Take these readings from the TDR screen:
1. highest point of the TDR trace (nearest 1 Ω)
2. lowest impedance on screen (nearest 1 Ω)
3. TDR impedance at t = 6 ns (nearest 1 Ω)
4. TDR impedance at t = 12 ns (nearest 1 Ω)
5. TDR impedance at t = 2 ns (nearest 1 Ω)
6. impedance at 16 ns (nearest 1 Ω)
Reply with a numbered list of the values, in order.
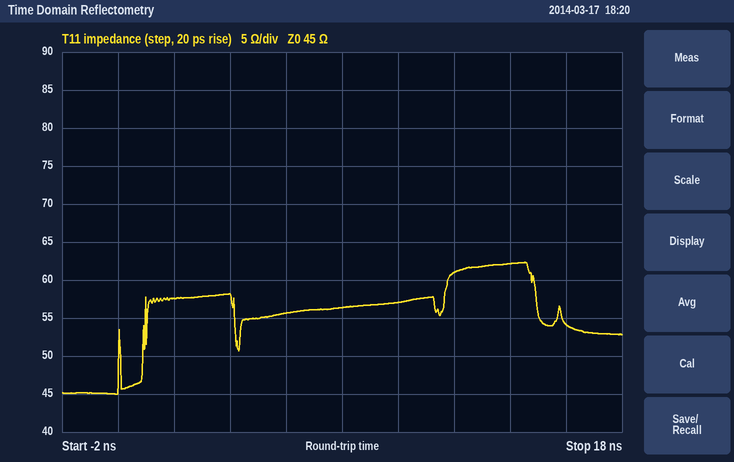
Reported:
1. 62 Ω
2. 45 Ω
3. 56 Ω
4. 61 Ω
5. 58 Ω
6. 54 Ω
